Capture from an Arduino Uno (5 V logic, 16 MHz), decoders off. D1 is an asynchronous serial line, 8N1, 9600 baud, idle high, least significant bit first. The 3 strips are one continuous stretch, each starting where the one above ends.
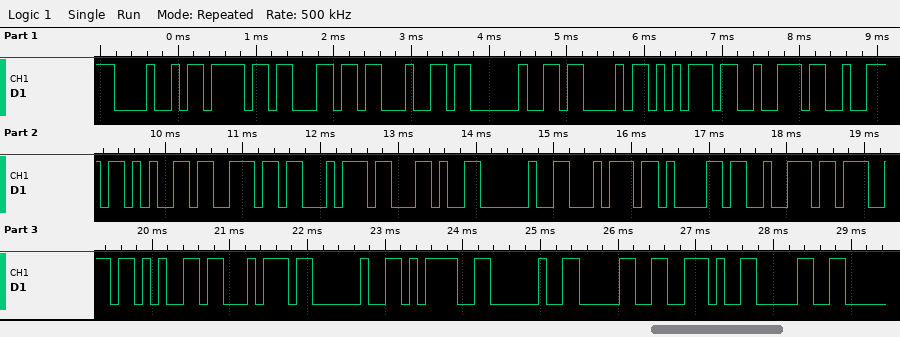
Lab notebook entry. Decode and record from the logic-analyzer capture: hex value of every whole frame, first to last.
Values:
48 6F 6C 64 20 43 75 72 72 65 6E 74 2C 20 74 61 72 67 65 74 20 3D 20 30 2E 30
